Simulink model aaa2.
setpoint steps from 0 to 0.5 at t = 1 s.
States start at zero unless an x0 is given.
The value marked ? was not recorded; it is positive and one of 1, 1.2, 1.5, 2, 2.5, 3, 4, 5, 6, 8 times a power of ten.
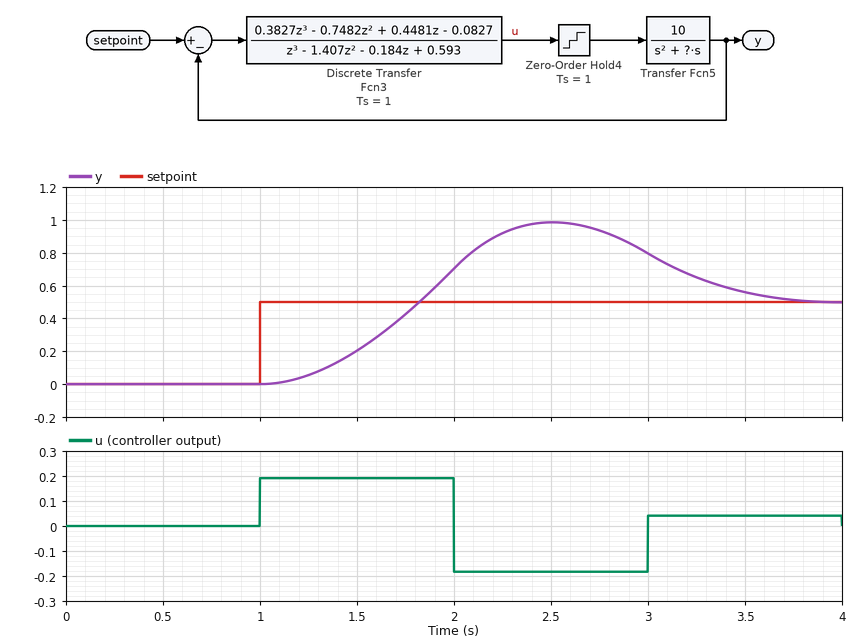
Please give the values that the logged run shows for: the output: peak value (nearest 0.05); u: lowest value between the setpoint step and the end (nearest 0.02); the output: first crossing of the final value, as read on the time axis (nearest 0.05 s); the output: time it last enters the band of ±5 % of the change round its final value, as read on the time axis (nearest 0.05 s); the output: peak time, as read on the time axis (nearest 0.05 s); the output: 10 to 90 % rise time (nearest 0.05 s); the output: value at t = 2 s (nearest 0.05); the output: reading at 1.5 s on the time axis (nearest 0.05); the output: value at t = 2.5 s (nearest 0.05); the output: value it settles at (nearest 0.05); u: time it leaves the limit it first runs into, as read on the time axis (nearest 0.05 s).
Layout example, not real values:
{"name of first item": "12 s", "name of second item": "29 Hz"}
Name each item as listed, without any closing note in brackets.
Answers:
{"the output: peak value": "1.00", "u: lowest value between the setpoint step and the end": "-0.18", "the output: first crossing of the final value, as read on the time axis": "1.80 s", "the output: time it last enters the band of ±5 % of the change round its final value, as read on the time axis": "3.65 s", "the output: peak time, as read on the time axis": "2.50 s", "the output: 10 to 90 % rise time": "0.55 s", "the output: value at t = 2 s": "0.70", "the output: reading at 1.5 s on the time axis": "0.20", "the output: value at t = 2.5 s": "1.00", "the output: value it settles at": "0.50", "u: time it leaves the limit it first runs into, as read on the time axis": "2.00 s"}
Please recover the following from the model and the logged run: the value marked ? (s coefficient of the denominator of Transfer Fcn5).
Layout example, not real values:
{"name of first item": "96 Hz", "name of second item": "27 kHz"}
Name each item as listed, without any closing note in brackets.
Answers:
{"the value marked ?": "1"}
